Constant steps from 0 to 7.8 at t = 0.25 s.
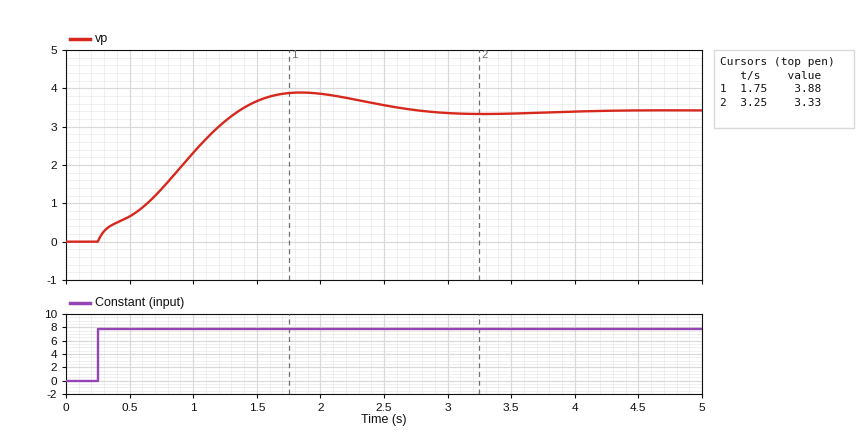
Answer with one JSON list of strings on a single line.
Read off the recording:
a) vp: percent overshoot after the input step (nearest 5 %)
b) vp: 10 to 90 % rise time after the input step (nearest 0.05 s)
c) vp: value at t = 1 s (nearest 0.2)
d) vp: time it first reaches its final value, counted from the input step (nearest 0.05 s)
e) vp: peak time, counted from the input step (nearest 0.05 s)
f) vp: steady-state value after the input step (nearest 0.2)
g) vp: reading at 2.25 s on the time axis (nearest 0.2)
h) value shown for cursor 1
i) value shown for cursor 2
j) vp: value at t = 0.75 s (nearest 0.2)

["15 %", "0.90 s", "2.4", "1.10 s", "1.60 s", "3.4", "3.8", "3.88", "3.33", "1.4"]
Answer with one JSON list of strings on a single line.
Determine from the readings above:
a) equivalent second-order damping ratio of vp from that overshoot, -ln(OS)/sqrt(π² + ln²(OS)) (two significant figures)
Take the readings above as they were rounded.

["0.52"]
